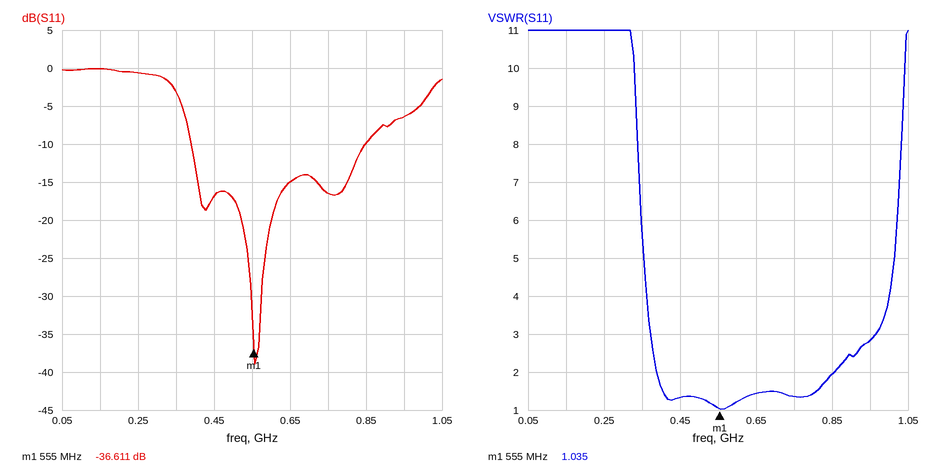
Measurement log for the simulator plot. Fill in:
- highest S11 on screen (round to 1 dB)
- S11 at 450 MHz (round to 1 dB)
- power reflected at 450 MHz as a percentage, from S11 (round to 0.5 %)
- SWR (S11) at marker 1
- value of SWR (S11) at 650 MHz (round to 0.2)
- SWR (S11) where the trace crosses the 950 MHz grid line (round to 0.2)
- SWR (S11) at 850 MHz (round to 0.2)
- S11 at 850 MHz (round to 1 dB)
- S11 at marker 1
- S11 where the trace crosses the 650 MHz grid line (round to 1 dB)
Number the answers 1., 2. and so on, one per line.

1. 0 dB
2. -17 dB
3. 2.0 %
4. 1.035
5. 1.4
6. 2.8
7. 2.0
8. -10 dB
9. -36.611 dB
10. -15 dB
